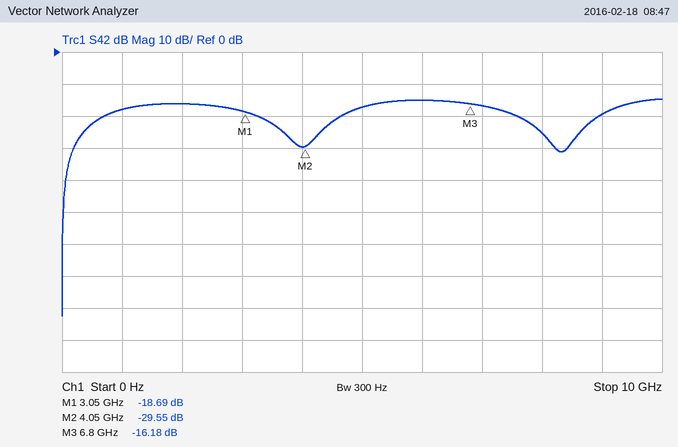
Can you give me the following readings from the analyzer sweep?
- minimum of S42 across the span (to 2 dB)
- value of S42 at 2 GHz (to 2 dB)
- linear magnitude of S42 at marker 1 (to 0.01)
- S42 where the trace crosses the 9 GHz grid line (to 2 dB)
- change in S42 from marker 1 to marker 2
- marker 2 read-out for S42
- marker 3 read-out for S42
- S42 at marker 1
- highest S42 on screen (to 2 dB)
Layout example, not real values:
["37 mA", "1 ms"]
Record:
["-82 dB", "-16 dB", "0.12", "-20 dB", "-10.86 dB", "-29.55 dB", "-16.18 dB", "-18.69 dB", "-14 dB"]
